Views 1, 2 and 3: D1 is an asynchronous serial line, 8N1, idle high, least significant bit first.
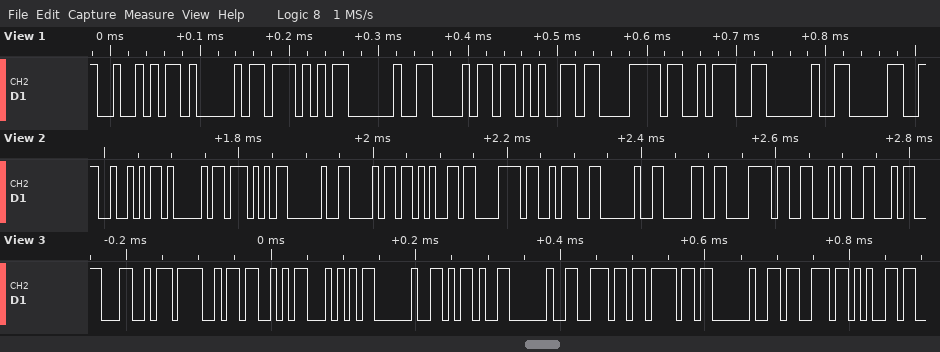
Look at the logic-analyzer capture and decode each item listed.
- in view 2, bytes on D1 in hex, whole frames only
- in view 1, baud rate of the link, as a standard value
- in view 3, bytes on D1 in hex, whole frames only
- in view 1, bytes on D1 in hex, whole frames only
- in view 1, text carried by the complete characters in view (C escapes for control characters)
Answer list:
52 41 57 20 68 65 78 3A 20 30 78 46 46
115200 baud
0x4C 0x4F 0x53 0x54 0x20 0x2D 0x20 0x6E 0x6F 0x20 0x73 0x65
52 41 57 20 68 65 78 3A 20 30
"RAW hex: 0"
